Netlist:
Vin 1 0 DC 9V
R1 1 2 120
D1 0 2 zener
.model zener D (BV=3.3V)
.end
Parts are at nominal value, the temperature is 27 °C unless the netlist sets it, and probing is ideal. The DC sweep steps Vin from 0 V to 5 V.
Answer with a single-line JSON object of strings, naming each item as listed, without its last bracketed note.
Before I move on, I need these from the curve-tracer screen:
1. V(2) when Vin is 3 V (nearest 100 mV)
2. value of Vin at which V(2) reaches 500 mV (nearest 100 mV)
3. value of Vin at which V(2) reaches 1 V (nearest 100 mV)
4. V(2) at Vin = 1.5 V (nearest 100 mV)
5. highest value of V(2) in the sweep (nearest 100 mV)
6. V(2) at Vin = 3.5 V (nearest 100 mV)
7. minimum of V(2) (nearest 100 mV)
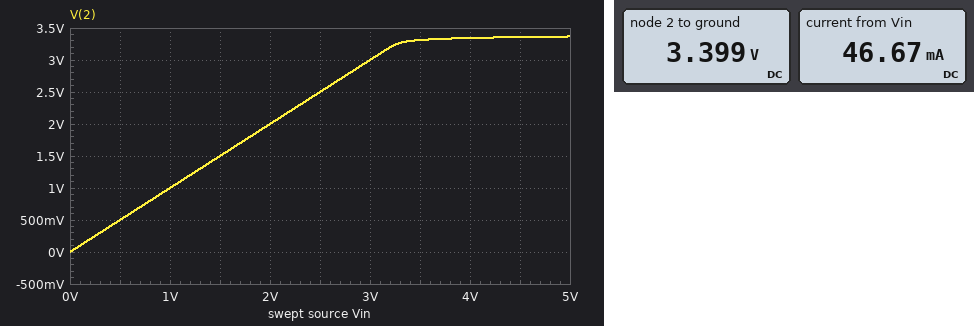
{"V(2) when Vin is 3 V": "3.0 V", "value of Vin at which V(2) reaches 500 mV": "500 mV", "value of Vin at which V(2) reaches 1 V": "1.0 V", "V(2) at Vin = 1.5 V": "1.5 V", "highest value of V(2) in the sweep": "3.4 V", "V(2) at Vin = 3.5 V": "3.3 V", "minimum of V(2)": "0 V"}
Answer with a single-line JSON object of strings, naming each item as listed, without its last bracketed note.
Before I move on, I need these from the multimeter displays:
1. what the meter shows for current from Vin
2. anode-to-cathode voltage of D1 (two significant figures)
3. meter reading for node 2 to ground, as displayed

{"what the meter shows for current from Vin": "46.67 mA", "anode-to-cathode voltage of D1": "-3.4 V", "meter reading for node 2 to ground, as displayed": "3.399 V"}
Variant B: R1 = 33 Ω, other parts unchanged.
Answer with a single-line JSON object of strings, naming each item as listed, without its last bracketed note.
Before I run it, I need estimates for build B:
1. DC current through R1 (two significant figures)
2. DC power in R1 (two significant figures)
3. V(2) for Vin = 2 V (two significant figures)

{"DC current through R1": "170 mA", "DC power in R1": "940 mW", "V(2) for Vin = 2 V": "2.0 V"}
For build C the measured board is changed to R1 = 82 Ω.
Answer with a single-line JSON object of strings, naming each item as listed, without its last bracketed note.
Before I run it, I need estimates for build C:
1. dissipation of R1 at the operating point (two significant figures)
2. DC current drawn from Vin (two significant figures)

{"dissipation of R1 at the operating point": "380 mW", "DC current drawn from Vin": "68 mA"}
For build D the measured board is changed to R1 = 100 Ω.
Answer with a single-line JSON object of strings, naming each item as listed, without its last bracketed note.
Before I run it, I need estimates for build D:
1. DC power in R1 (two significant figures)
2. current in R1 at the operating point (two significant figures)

{"DC power in R1": "310 mW", "current in R1 at the operating point": "56 mA"}
